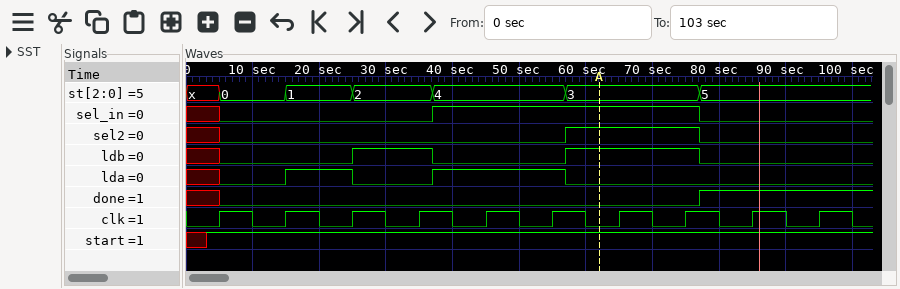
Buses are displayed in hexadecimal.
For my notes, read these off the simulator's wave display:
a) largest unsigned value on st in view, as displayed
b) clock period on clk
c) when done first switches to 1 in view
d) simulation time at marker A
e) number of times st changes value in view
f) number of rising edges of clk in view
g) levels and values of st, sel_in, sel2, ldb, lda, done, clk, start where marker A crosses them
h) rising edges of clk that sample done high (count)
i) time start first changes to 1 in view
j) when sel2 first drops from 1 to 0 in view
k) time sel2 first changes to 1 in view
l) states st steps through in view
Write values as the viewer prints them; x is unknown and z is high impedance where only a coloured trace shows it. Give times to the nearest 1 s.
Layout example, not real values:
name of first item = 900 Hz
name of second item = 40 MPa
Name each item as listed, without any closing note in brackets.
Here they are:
largest unsigned value on st in view, as displayed = 5
clock period on clk = 10 s
when done first switches to 1 in view = 77 s
simulation time at marker A = 62 s
number of times st changes value in view = 6
number of rising edges of clk in view = 10
levels and values of st, sel_in, sel2, ldb, lda, done, clk, start where marker A crosses them = st=3, sel_in=1, sel2=1, ldb=1, lda=0, done=0, clk=0, start=1
rising edges of clk that sample done high = 2
time start first changes to 1 in view = 3 s
when sel2 first drops from 1 to 0 in view = 77 s
time sel2 first changes to 1 in view = 57 s
states st steps through in view = x, 0, 1, 2, 4, 3, 5
